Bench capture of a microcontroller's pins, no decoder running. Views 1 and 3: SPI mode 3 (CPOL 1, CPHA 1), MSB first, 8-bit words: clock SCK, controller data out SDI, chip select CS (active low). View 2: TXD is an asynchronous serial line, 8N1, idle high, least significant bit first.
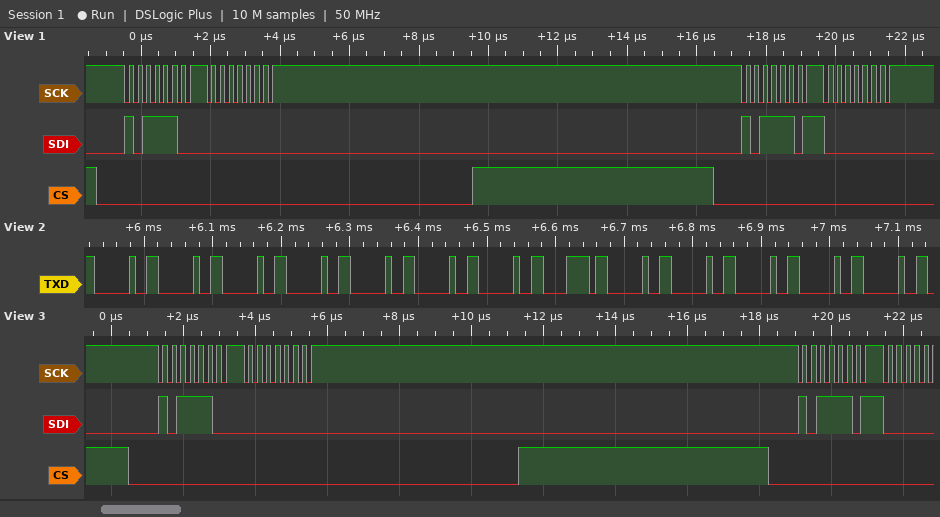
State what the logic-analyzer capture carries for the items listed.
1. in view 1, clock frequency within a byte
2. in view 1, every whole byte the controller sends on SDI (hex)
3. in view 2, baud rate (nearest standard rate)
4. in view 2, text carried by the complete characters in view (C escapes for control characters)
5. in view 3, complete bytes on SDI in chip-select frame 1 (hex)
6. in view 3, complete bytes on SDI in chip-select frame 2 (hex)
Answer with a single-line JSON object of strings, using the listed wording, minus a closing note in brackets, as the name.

{"in view 1, clock frequency within a byte": "4 MHz", "in view 1, every whole byte the controller sends on SDI": "BC 00 BD 00", "in view 2, baud rate": "115200 baud", "in view 2, text carried by the complete characters in view": "\"       x     \"", "in view 3, complete bytes on SDI in chip-select frame 1": "BC 00", "in view 3, complete bytes on SDI in chip-select frame 2": "BD"}
